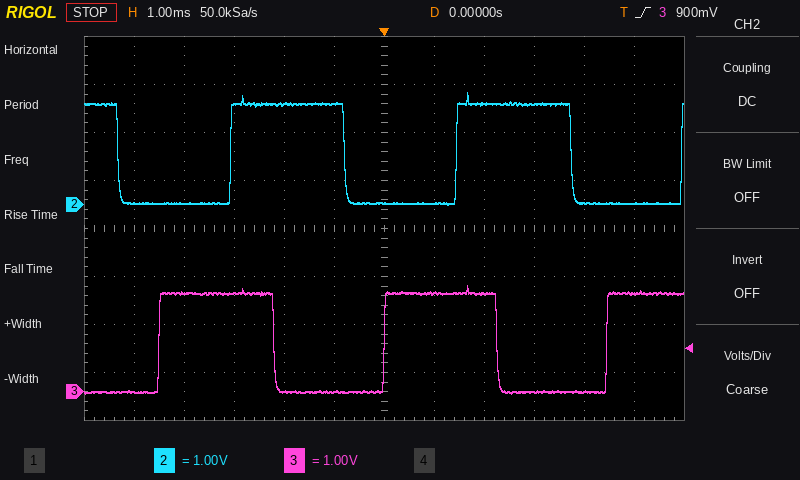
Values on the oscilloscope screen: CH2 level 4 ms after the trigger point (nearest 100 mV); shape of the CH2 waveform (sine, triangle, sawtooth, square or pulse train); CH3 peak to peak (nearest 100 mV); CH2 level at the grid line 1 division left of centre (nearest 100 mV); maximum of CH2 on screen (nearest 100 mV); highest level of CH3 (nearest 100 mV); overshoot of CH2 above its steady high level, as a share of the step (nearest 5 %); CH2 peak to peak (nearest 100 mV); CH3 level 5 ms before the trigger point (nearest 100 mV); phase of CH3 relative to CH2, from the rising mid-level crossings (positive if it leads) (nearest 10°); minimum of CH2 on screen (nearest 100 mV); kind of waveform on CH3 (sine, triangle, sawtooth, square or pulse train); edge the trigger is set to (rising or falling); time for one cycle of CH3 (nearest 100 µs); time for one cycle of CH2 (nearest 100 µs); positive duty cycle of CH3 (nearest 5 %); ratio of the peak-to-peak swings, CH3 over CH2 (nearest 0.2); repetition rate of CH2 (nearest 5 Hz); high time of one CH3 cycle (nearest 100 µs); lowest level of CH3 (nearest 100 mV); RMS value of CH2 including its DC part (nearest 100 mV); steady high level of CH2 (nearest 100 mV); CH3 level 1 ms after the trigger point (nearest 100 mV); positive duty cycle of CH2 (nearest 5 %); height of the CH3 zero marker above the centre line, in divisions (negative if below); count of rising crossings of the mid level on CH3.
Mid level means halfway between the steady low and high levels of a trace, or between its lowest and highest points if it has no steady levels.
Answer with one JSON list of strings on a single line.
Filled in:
["0.0 V", "square", "2.2 V", "2.1 V", "2.3 V", "2.2 V", "10 %", "2.3 V", "0.0 V", "+120°", "0.0 V", "square", "rising", "4.5 ms", "4.5 ms", "50 %", "1.0", "220 Hz", "2.3 ms", "0.0 V", "1.5 V", "2.1 V", "2.1 V", "50 %", "-3.4 div", "3"]
